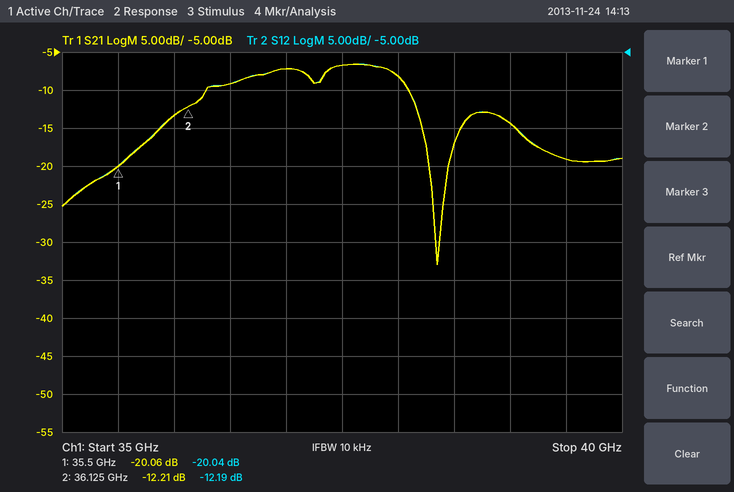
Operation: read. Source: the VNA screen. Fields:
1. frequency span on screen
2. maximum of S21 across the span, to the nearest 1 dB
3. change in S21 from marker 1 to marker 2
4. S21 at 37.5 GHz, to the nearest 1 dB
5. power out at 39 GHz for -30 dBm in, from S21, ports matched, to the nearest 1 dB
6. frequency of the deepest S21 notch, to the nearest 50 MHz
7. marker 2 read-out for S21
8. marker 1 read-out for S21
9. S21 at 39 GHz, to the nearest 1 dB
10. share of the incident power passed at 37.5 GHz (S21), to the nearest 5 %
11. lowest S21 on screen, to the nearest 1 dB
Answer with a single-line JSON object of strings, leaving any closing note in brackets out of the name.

{"frequency span on screen": "5 GHz", "maximum of S21 across the span, to the nearest 1 dB": "-7 dB", "change in S21 from marker 1 to marker 2": "7.85 dB", "S21 at 37.5 GHz, to the nearest 1 dB": "-7 dB", "power out at 39 GHz for -30 dBm in, from S21, ports matched, to the nearest 1 dB": "-44 dBm", "frequency of the deepest S21 notch, to the nearest 50 MHz": "38.35 GHz", "marker 2 read-out for S21": "-12.21 dB", "marker 1 read-out for S21": "-20.06 dB", "S21 at 39 GHz, to the nearest 1 dB": "-14 dB", "share of the incident power passed at 37.5 GHz (S21), to the nearest 5 %": "20 %", "lowest S21 on screen, to the nearest 1 dB": "-33 dB"}
